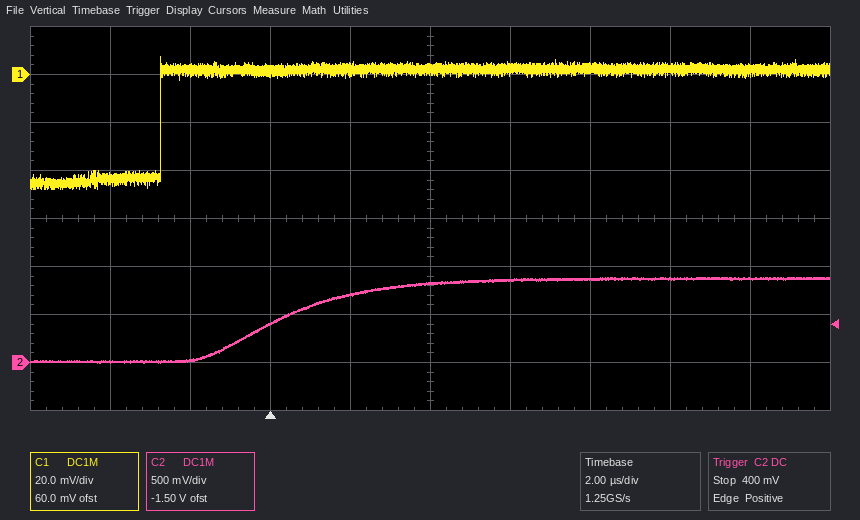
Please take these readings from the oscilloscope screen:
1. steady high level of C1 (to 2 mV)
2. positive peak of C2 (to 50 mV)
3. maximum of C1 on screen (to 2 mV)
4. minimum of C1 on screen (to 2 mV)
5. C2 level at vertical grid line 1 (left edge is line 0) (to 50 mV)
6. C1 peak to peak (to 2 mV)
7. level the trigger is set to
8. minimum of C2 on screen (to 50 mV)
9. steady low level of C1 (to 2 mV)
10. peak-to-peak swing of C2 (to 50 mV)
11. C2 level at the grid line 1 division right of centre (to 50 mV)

2 mV
900 mV
8 mV
-48 mV
0 mV
56 mV
400 mV
0 mV
-44 mV
900 mV
850 mV
